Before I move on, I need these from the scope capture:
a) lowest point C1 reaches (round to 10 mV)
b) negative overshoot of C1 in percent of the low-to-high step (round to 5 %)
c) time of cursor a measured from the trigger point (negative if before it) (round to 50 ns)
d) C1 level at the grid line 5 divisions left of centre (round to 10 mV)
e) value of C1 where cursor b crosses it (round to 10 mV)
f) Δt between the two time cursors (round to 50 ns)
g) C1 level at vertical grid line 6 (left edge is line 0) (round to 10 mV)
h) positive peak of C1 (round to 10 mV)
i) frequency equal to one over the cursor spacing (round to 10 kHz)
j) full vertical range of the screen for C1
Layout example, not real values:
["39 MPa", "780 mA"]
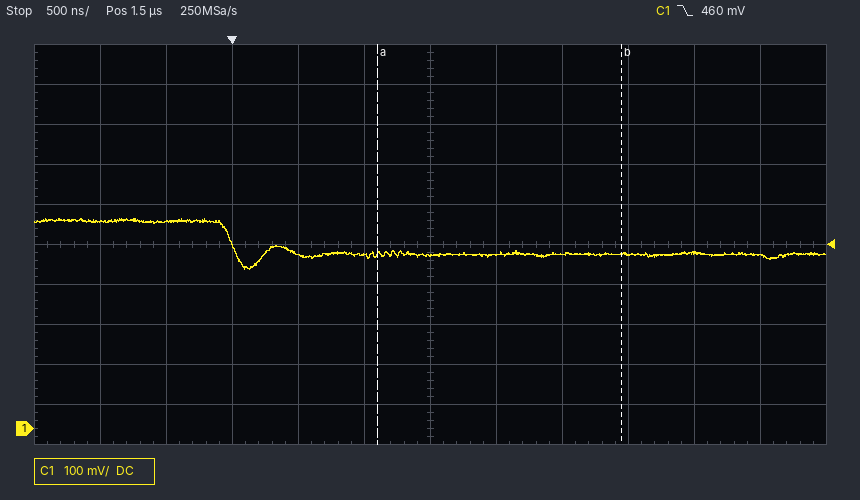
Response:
["400 mV", "45 %", "+1.10 µs", "520 mV", "440 mV", "1.85 µs", "430 mV", "520 mV", "540 kHz", "1 V"]
